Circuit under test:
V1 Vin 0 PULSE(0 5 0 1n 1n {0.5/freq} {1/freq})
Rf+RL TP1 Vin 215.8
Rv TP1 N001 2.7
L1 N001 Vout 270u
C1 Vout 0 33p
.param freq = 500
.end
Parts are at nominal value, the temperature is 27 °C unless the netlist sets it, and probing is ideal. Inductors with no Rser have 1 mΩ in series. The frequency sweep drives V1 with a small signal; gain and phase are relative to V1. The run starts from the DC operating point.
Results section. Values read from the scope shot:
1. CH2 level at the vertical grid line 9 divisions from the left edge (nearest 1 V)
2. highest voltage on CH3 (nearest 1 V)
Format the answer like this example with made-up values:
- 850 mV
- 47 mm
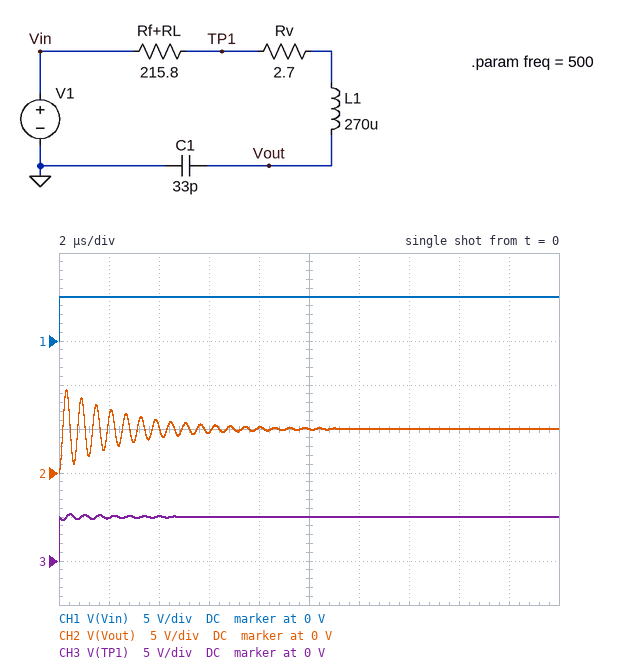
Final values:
- 5 V
- 5 V
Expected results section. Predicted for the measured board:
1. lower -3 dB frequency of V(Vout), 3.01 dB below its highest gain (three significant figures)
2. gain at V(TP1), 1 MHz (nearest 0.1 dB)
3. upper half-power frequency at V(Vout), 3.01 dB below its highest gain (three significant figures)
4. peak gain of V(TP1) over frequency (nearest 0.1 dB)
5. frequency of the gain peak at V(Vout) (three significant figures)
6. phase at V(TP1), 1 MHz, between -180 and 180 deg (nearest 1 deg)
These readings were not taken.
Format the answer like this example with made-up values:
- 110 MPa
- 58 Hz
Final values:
- 1.62 MHz
- 0 dB
- 1.75 MHz
- 0 dB
- 1.68 MHz
- -4 deg
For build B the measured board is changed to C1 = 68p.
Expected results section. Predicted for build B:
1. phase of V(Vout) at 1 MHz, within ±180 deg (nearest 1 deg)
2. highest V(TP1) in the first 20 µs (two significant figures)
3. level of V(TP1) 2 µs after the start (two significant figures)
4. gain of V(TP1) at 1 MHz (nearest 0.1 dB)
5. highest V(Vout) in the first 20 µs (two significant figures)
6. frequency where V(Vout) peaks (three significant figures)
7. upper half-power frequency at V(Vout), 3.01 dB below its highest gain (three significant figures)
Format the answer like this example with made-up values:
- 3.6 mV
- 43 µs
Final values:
- -19 deg
- 5.4 V
- 4.8 V
- -0.5 dB
- 9.2 V
- 1.17 MHz
- 1.23 MHz
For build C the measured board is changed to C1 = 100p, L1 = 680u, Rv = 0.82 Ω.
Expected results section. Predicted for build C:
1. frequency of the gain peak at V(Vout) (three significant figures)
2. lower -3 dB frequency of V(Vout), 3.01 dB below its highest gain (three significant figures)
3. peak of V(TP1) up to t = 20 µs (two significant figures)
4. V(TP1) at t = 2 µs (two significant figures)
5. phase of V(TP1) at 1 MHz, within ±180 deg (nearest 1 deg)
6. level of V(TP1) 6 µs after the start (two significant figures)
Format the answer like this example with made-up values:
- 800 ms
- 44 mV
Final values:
- 609 kHz
- 583 kHz
- 5.3 V
- 4.7 V
- 5 deg
- 5.1 V
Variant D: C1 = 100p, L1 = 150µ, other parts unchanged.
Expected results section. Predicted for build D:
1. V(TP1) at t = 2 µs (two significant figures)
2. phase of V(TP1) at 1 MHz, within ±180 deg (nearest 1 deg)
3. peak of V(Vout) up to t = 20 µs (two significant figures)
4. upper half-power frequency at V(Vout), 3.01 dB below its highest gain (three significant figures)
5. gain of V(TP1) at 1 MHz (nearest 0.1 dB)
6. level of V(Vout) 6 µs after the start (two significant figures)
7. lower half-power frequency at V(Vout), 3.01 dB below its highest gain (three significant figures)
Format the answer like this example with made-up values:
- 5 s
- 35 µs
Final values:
- 5.1 V
- -18 deg
- 8.8 V
- 1.40 MHz
- -0.5 dB
- 5.0 V
- 1.17 MHz
